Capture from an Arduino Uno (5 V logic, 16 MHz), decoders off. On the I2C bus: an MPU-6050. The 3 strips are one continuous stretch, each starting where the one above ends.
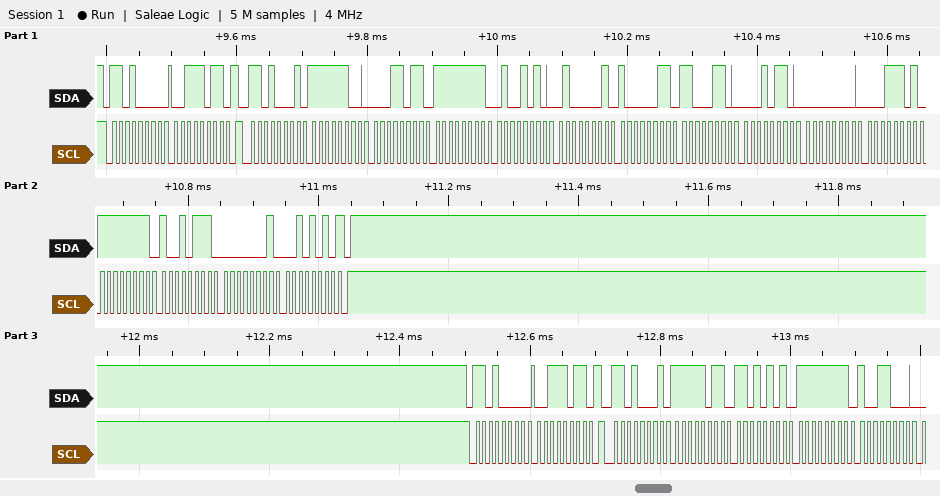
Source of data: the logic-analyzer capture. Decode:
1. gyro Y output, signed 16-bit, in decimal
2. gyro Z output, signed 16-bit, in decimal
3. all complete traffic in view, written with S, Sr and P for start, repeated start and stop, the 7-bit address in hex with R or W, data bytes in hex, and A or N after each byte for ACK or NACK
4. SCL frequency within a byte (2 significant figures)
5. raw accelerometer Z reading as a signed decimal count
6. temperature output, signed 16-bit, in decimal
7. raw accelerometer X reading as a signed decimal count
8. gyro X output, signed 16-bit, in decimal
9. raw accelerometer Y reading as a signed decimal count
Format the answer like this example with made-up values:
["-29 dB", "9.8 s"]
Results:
["-105", "298", "S 68W A 3B A Sr 68R A FC A 1B A FF A 4A A 41 A 83 A C6 A 16 A 00 A 1D A FF A 97 A 01 A 2A N P S 68W A 3B A Sr 68R A FB A D5 A FF A 98 A", "100 kHz", "16771", "-14826", "-997", "29", "-182"]
